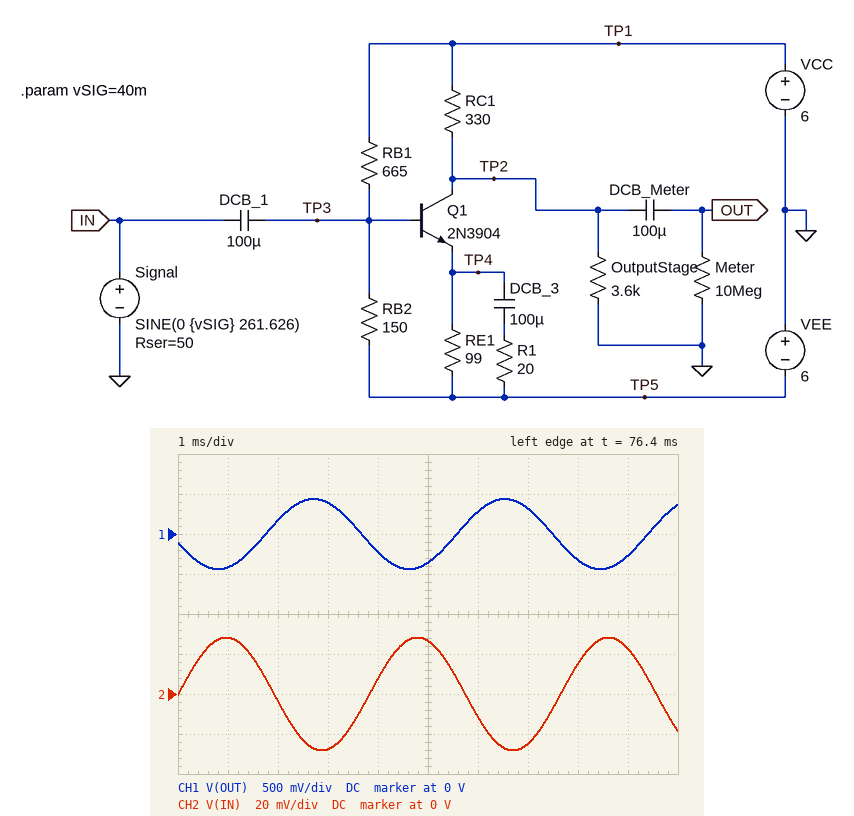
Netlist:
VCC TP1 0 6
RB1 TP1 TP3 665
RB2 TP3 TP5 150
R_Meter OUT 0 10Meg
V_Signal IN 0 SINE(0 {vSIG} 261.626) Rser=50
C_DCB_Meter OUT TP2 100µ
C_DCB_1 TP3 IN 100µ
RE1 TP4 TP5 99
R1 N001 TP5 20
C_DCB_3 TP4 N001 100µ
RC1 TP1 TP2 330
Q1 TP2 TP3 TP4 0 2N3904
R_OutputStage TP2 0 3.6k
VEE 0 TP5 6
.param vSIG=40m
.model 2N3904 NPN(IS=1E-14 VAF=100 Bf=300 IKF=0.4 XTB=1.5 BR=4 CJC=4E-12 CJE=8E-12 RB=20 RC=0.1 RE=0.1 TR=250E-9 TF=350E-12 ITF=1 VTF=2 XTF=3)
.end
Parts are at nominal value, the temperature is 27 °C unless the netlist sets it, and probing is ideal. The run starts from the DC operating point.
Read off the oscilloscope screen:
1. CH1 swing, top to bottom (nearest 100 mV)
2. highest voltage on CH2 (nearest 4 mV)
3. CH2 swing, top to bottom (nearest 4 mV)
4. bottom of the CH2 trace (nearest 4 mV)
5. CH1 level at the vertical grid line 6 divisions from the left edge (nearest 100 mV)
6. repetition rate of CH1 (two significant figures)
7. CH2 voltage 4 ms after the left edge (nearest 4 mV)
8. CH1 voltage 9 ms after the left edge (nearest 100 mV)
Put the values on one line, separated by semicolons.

900 mV; 28 mV; 56 mV; -28 mV; 300 mV; 260 Hz; 8 mV; -300 mV
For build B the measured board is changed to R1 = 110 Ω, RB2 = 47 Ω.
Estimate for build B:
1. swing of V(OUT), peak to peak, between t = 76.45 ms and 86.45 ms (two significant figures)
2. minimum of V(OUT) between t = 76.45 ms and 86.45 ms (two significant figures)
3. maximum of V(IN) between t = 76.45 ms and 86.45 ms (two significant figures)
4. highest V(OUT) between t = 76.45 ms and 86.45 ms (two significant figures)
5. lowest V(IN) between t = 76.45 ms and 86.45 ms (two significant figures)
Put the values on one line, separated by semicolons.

160 mV; -80 mV; 19 mV; 76 mV; -19 mV
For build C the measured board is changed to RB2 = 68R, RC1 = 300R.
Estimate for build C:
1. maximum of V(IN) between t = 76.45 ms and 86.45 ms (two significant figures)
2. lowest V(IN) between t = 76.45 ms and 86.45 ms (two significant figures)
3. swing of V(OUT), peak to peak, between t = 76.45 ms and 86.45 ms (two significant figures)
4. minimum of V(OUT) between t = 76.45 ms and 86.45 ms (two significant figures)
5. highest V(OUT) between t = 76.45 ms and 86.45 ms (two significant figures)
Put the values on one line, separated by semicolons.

22 mV; -22 mV; 510 mV; -260 mV; 250 mV
